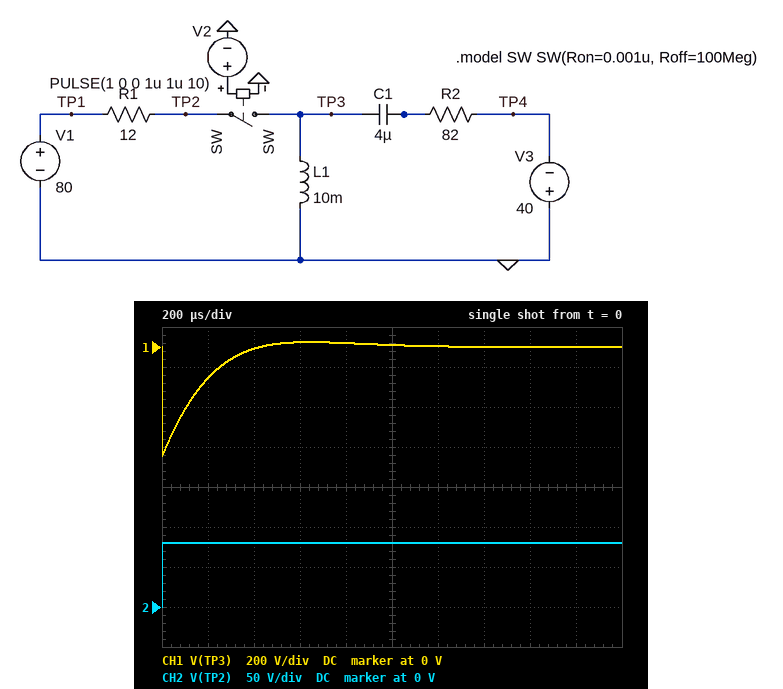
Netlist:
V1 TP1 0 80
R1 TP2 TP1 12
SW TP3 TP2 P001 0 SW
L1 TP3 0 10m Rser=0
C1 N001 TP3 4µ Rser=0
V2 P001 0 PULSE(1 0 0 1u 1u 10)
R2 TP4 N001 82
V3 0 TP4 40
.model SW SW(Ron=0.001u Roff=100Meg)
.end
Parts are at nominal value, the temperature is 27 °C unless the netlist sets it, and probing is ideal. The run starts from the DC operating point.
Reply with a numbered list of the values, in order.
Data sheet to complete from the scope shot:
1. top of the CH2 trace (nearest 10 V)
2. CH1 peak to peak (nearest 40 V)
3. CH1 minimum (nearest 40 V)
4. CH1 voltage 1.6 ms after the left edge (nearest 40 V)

1. 80 V
2. 560 V
3. -560 V
4. 0 V
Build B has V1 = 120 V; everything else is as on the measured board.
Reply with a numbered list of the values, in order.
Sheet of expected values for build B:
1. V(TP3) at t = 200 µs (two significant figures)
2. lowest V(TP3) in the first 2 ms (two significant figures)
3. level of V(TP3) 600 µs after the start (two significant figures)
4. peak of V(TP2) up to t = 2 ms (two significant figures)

1. -230 V
2. -820 V
3. 36 V
4. 120 V
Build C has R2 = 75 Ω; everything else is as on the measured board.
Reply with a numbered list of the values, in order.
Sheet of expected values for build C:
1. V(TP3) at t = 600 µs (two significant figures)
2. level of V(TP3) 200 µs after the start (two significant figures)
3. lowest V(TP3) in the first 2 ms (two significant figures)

1. 27 V
2. -170 V
3. -500 V
